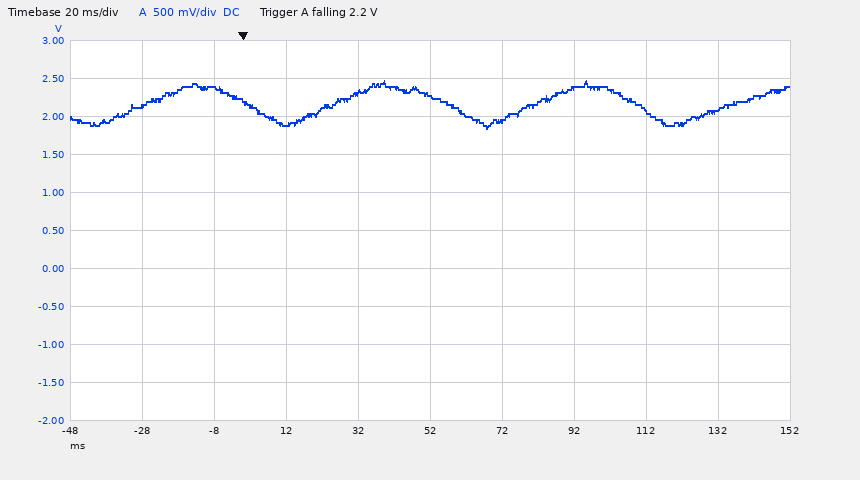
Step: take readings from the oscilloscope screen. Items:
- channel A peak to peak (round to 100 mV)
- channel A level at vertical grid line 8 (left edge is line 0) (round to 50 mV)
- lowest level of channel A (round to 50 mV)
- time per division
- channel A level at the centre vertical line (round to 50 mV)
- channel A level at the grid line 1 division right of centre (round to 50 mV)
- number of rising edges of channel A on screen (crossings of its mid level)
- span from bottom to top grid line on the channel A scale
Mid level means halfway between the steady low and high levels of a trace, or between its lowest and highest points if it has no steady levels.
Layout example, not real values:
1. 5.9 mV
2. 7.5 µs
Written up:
1. 600 mV
2. 2.10 V
3. 1.85 V
4. 20 ms
5. 2.30 V
6. 1.95 V
7. 4
8. 5 V
